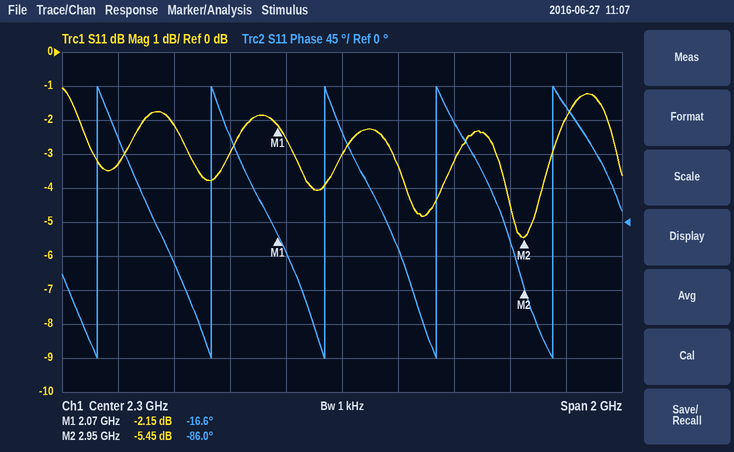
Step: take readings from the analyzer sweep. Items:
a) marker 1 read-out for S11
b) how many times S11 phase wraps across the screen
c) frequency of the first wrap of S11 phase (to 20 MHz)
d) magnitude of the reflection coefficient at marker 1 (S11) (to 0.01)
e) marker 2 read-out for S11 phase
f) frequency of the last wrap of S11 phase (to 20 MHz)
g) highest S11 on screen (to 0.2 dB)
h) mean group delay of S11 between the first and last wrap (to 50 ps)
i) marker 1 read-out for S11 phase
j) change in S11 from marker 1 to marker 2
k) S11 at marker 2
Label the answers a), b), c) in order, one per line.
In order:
a) -2.15 dB
b) 5
c) 1.42 GHz
d) 0.78
e) -86.0°
f) 3.06 GHz
g) -1.0 dB
h) 2.45 ns
i) -16.6°
j) -3.30 dB
k) -5.45 dB
